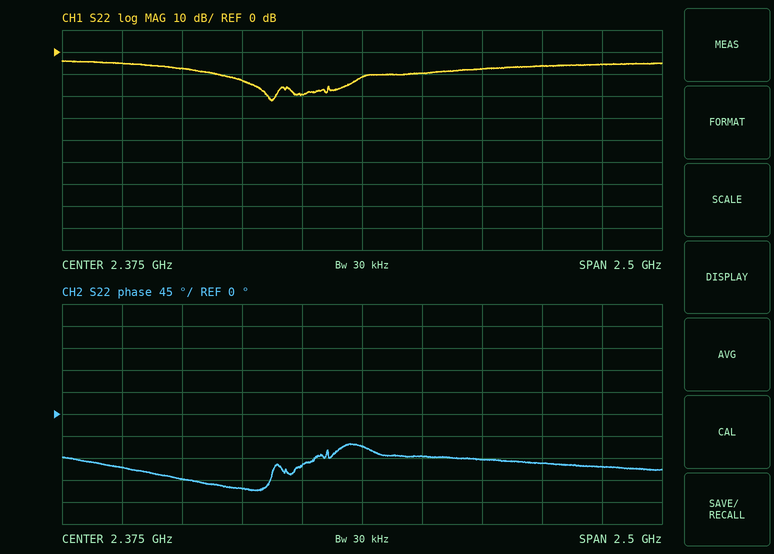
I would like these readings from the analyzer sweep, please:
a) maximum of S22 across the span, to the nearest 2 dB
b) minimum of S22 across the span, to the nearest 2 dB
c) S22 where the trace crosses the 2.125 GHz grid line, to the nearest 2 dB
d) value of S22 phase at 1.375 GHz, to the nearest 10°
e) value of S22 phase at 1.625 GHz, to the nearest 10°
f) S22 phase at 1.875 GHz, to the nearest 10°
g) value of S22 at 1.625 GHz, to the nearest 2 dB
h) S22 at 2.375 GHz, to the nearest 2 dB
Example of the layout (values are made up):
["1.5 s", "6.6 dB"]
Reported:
["-4 dB", "-22 dB", "-20 dB", "-110°", "-130°", "-150°", "-8 dB", "-12 dB"]
